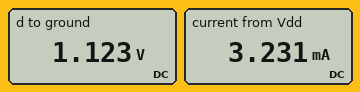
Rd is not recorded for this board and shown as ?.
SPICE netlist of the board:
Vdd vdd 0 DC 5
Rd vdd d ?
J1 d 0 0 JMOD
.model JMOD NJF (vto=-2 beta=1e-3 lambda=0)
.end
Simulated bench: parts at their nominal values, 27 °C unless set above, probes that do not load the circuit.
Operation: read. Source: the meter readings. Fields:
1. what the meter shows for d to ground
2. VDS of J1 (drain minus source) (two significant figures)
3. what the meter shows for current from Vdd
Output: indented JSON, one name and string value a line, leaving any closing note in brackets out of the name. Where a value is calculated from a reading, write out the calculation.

{
  "what the meter shows for d to ground": "1.123 V",
  "VDS of J1 (drain minus source)": "1.123 V = 1.1 V",
  "what the meter shows for current from Vdd": "3.231 mA"
}
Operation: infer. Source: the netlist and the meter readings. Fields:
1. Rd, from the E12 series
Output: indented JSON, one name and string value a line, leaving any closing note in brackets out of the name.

{
  "Rd, from the E12 series": "1.2 kΩ"
}
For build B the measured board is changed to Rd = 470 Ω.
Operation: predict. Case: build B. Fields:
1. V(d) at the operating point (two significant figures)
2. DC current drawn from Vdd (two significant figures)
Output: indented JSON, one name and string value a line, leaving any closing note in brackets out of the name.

{
  "V(d) at the operating point": "3.1 V",
  "DC current drawn from Vdd": "4.0 mA"
}
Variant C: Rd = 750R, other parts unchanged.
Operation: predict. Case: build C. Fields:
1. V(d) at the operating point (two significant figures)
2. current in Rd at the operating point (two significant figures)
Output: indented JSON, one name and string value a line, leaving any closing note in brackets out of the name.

{
  "V(d) at the operating point": "2.0 V",
  "current in Rd at the operating point": "4.0 mA"
}
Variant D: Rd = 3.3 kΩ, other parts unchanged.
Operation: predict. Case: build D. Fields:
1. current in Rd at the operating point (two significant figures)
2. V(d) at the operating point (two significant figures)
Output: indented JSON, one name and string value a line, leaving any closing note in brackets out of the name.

{
  "current in Rd at the operating point": "1.4 mA",
  "V(d) at the operating point": "390 mV"
}
